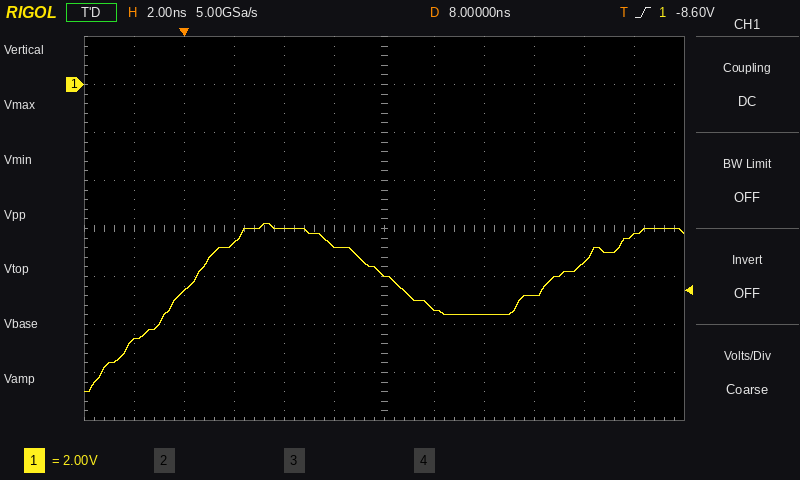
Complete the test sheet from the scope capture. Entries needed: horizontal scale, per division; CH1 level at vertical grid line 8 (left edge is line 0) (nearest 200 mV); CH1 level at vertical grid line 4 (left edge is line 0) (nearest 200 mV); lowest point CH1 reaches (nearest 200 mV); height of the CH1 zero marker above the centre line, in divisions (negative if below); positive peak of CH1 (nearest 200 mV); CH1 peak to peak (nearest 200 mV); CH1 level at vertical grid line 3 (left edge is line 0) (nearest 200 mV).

2 ns
-9.6 V
-6.0 V
-12.8 V
+3.0 div
-5.8 V
7.0 V
-6.6 V
